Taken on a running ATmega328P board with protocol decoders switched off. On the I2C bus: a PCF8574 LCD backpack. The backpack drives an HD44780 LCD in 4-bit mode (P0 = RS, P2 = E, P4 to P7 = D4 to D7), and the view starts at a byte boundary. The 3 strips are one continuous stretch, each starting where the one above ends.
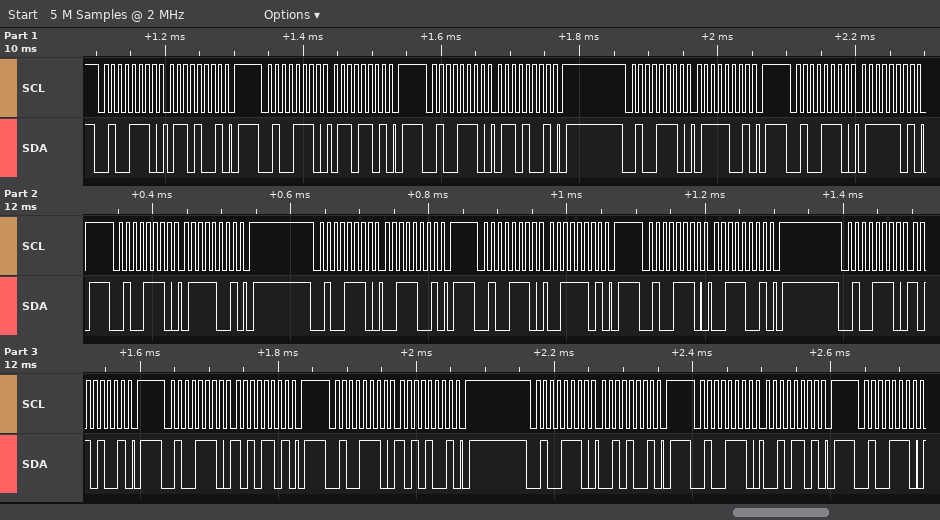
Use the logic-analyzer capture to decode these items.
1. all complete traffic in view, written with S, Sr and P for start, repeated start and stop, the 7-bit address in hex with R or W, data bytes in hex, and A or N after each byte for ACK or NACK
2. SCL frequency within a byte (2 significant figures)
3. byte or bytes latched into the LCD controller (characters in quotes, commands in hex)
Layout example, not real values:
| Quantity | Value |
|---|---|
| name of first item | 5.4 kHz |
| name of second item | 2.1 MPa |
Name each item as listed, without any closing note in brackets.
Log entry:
| Quantity | Value |
|---|---|
| all complete traffic in view, written with S, Sr and P for start, repeated start and stop, the 7-bit address in hex with R or W, data bytes in hex, and A or N after each byte for ACK or NACK | S 27W A 69 A P S 27W A 6D A P S 27W A 69 A P S 27W A 79 A P S 27W A 7D A P S 27W A 79 A P S 27W A 39 A P S 27W A 3D A P S 27W A 39 A P S 27W A A9 A P S 27W A AD A P S 27W A A9 A P S 27W A 29 A P S 27W A 2D A P S 27W A |
| SCL frequency within a byte | 100 kHz |
| byte or bytes latched into the LCD controller | 'g' ':' |
